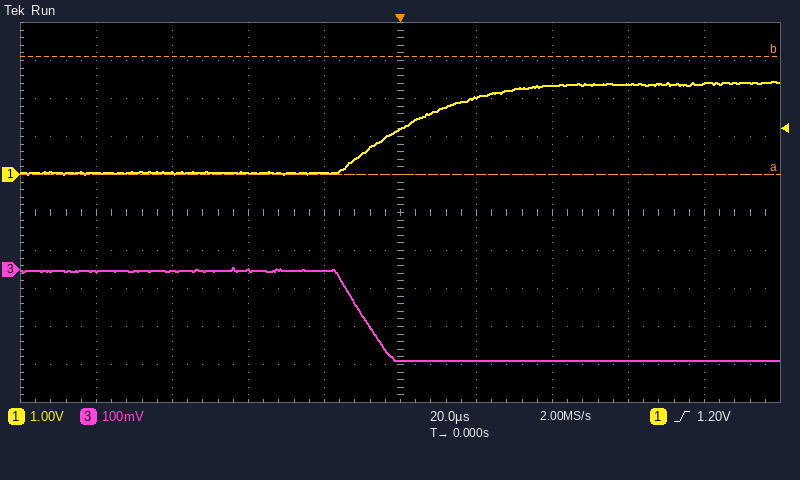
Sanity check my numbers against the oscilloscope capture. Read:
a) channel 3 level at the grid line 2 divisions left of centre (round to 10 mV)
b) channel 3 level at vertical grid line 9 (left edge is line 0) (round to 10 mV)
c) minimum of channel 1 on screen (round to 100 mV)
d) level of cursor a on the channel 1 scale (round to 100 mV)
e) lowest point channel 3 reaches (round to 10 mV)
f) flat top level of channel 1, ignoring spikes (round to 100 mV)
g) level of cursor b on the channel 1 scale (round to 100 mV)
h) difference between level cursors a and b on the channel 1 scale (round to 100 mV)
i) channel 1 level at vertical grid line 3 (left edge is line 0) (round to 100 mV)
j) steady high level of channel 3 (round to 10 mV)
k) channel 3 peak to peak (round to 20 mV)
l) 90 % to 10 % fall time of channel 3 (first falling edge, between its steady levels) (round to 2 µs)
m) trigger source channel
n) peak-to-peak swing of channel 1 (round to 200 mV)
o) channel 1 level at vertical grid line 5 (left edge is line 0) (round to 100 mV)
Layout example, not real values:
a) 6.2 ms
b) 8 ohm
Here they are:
a) 0 mV
b) -240 mV
c) 0.0 V
d) 0.0 V
e) -240 mV
f) 2.4 V
g) 3.1 V
h) 3.1 V
i) 0.0 V
j) 0 mV
k) 240 mV
l) 12 µs
m) channel 1
n) 2.4 V
o) 1.2 V
